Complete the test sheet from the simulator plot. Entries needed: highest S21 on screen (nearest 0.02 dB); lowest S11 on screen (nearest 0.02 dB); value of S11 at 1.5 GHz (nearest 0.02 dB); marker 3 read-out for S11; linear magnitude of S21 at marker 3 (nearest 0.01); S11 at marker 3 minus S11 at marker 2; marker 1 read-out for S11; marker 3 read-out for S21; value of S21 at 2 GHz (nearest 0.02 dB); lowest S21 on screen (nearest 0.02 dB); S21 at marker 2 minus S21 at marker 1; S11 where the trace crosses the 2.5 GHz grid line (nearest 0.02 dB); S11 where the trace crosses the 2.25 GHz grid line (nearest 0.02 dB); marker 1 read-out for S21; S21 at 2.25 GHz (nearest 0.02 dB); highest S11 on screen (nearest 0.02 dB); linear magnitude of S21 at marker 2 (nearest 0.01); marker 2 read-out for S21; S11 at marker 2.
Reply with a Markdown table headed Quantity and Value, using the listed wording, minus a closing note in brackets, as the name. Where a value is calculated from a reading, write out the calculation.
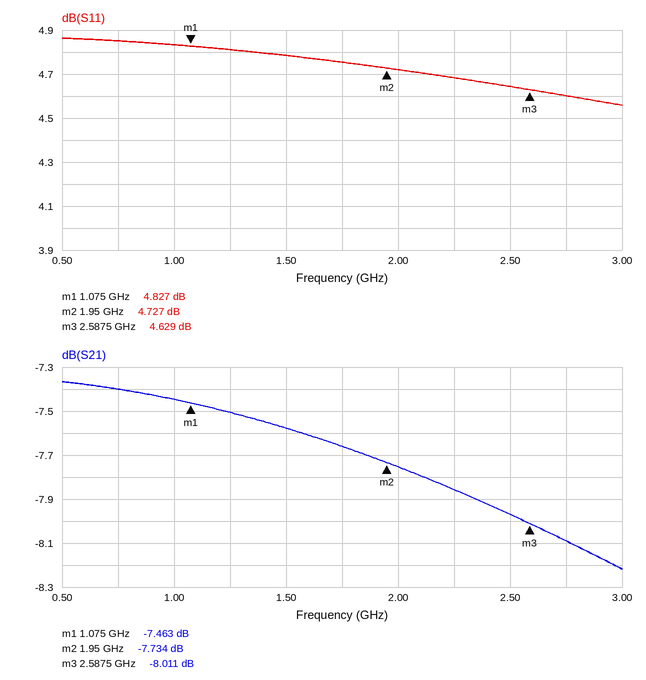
| Quantity | Value |
|---|---|
| highest S21 on screen | -7.36 dB |
| lowest S11 on screen | 4.56 dB |
| value of S11 at 1.5 GHz | 4.78 dB |
| marker 3 read-out for S11 | 4.629 dB |
| linear magnitude of S21 at marker 3 | 10^(-8.011/20) ≈ 0.40 |
| S11 at marker 3 minus S11 at marker 2 | 4.629 − (4.727) = -0.098 dB |
| marker 1 read-out for S11 | 4.827 dB |
| marker 3 read-out for S21 | -8.011 dB |
| value of S21 at 2 GHz | -7.76 dB |
| lowest S21 on screen | -8.22 dB |
| S21 at marker 2 minus S21 at marker 1 | -7.734 − (-7.463) = -0.271 dB |
| S11 where the trace crosses the 2.5 GHz grid line | 4.64 dB |
| S11 where the trace crosses the 2.25 GHz grid line | 4.68 dB |
| marker 1 read-out for S21 | -7.463 dB |
| S21 at 2.25 GHz | -7.86 dB |
| highest S11 on screen | 4.86 dB |
| linear magnitude of S21 at marker 2 | 10^(-7.734/20) ≈ 0.41 |
| marker 2 read-out for S21 | -7.734 dB |
| S11 at marker 2 | 4.727 dB |
